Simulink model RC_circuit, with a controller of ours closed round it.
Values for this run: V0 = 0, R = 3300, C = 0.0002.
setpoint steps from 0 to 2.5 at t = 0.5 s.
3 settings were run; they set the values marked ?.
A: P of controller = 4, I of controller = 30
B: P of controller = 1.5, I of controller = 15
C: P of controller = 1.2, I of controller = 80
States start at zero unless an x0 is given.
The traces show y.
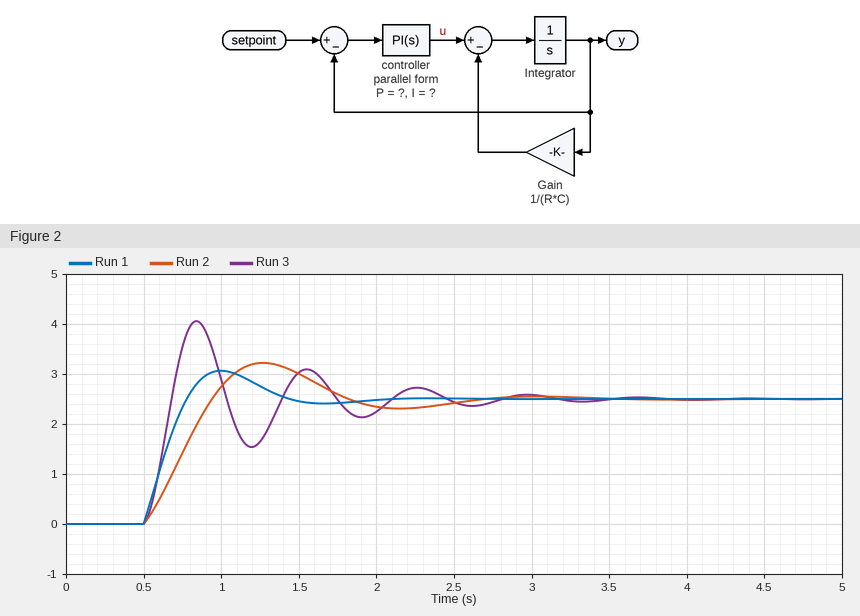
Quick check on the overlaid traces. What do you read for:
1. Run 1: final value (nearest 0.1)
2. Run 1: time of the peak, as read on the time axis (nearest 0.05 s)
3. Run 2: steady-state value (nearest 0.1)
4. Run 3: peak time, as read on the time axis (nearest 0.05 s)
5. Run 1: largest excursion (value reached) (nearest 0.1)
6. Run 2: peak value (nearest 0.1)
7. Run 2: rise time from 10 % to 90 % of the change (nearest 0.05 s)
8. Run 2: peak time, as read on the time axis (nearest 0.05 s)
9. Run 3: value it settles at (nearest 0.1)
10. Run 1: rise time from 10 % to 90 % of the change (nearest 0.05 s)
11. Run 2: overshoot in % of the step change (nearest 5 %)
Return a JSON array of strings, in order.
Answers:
["2.5", "1.00 s", "2.5", "0.85 s", "3.1", "3.2", "0.35 s", "1.25 s", "2.5", "0.20 s", "30 %"]
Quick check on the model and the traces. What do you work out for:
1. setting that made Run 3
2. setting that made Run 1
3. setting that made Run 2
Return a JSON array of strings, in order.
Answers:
["C", "A", "B"]
